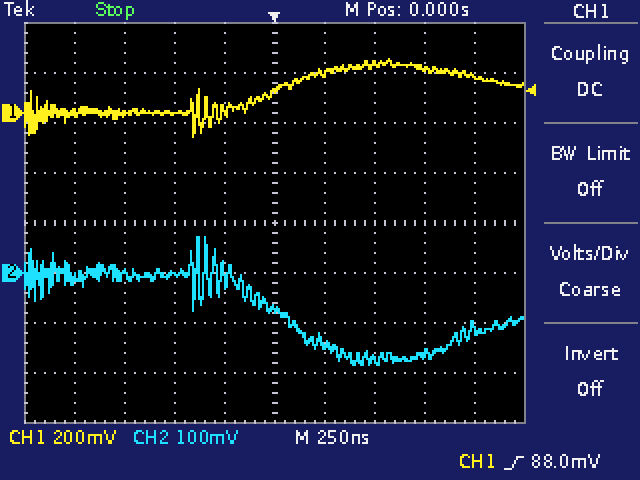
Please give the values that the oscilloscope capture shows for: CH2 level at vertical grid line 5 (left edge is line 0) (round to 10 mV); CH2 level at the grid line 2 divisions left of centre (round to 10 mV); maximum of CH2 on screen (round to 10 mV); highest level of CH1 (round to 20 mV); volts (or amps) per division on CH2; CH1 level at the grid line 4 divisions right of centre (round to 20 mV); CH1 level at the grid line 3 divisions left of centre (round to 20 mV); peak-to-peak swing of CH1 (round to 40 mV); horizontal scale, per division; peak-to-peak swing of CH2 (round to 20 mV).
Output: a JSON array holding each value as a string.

["-70 mV", "0 mV", "70 mV", "220 mV", "100 mV", "140 mV", "0 mV", "320 mV", "250 ns", "260 mV"]
